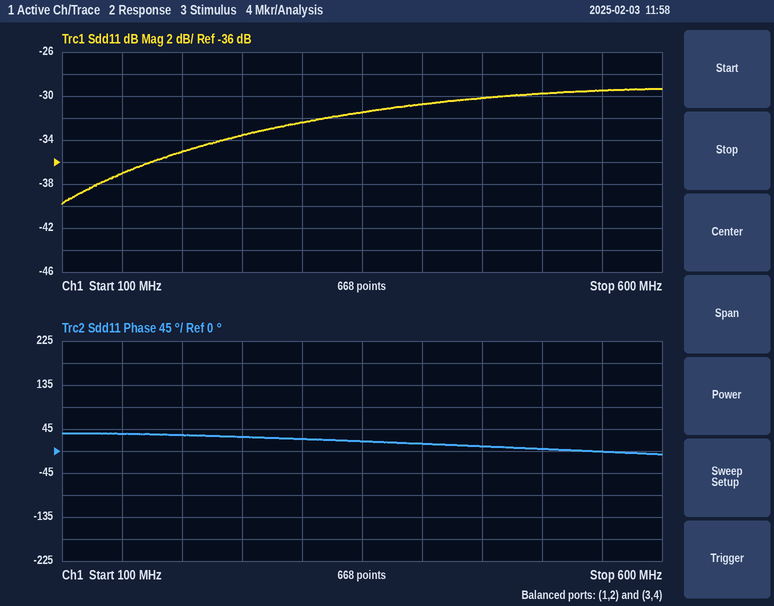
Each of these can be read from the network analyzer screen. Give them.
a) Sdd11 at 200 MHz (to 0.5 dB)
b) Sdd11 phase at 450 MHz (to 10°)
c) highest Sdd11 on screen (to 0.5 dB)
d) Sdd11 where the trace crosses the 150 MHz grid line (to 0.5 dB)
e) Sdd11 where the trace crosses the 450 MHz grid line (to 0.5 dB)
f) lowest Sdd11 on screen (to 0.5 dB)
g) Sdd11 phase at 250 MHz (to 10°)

-35.0 dB
10°
-29.5 dB
-37.0 dB
-30.0 dB
-40.0 dB
30°
